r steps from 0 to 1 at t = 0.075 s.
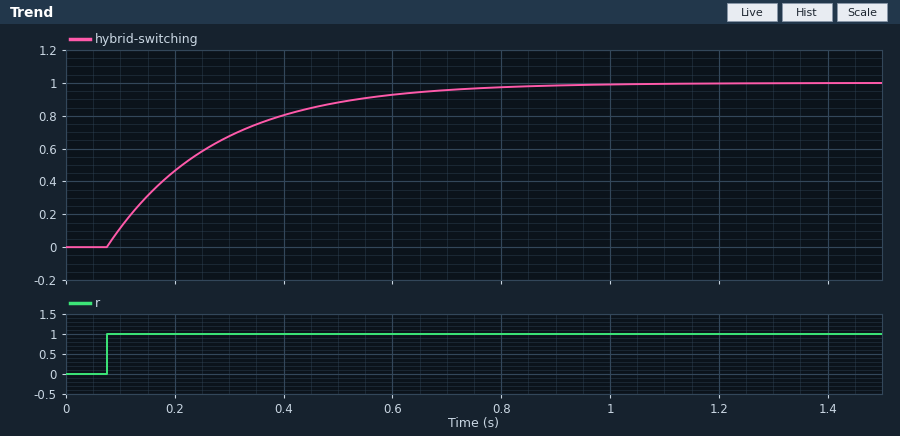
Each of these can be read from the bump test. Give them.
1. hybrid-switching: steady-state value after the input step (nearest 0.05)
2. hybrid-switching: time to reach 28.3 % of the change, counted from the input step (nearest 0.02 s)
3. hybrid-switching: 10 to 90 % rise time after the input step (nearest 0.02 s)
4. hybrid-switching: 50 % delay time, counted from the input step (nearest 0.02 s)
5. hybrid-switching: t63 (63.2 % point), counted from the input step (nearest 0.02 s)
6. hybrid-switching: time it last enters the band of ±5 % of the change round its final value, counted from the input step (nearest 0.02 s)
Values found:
1.00
0.06 s
0.44 s
0.14 s
0.20 s
0.60 s
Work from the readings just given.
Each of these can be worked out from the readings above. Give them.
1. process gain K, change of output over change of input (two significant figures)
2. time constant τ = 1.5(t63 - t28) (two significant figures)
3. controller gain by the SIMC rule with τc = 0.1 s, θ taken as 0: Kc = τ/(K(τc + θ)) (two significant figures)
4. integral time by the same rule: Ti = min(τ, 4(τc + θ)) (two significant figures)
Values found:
1.0
0.21 s
2.1
0.21 s
